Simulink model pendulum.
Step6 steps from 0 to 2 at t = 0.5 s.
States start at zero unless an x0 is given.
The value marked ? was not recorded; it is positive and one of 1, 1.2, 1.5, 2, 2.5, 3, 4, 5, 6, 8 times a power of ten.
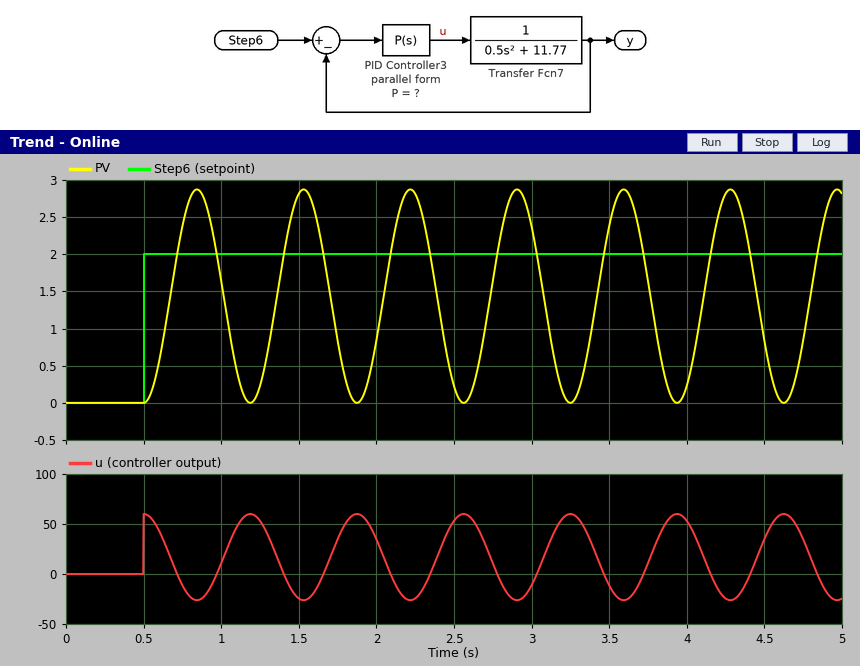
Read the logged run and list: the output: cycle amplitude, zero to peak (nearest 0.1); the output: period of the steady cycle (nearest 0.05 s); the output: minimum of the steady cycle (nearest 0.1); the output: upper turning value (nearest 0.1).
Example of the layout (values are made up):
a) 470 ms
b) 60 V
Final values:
a) 1.4
b) 0.70 s
c) 0.0
d) 2.9
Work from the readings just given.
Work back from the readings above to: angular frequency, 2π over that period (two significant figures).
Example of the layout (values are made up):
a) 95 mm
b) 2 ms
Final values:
a) 9.0 rad/s
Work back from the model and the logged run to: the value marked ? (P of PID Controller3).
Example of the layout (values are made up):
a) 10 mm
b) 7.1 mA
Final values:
a) 30
